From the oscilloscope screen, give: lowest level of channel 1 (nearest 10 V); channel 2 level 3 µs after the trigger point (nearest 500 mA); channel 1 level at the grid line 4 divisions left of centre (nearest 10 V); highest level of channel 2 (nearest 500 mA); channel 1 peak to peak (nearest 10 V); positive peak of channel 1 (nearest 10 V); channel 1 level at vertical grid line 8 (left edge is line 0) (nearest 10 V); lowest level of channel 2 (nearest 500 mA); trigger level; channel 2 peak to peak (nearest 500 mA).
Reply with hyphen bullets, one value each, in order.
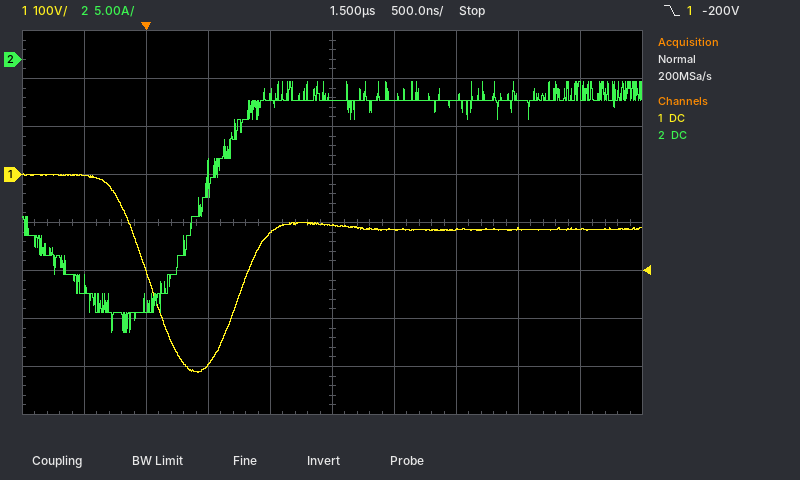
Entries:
- -410 V
- -4.0 A
- 0 V
- -2.5 A
- 410 V
- 0 V
- -110 V
- -28.5 A
- -200 V
- 26.0 A
